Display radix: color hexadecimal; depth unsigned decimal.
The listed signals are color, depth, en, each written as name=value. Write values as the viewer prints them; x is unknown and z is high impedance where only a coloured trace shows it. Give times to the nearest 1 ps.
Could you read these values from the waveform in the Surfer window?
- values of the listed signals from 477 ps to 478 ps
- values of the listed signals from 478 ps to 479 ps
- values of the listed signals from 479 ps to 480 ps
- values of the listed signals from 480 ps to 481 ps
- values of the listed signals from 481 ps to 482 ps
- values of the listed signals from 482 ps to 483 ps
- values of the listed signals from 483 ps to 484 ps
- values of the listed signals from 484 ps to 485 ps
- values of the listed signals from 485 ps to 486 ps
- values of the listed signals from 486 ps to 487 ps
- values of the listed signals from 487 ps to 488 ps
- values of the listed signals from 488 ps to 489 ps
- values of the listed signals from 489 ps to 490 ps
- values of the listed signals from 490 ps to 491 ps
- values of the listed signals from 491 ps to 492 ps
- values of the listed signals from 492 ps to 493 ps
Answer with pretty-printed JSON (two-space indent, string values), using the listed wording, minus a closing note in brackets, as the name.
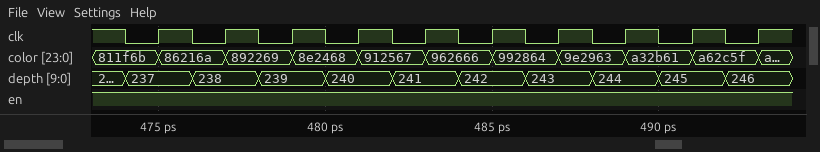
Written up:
{
  "values of the listed signals from 477 ps to 478 ps": "color=892269, depth=238, en=1",
  "values of the listed signals from 478 ps to 479 ps": "color=892269, depth=239, en=1",
  "values of the listed signals from 479 ps to 480 ps": "color=8e2468, depth=239, en=1",
  "values of the listed signals from 480 ps to 481 ps": "color=8e2468, depth=240, en=1",
  "values of the listed signals from 481 ps to 482 ps": "color=912567, depth=240, en=1",
  "values of the listed signals from 482 ps to 483 ps": "color=912567, depth=241, en=1",
  "values of the listed signals from 483 ps to 484 ps": "color=962666, depth=241, en=1",
  "values of the listed signals from 484 ps to 485 ps": "color=962666, depth=242, en=1",
  "values of the listed signals from 485 ps to 486 ps": "color=992864, depth=242, en=1",
  "values of the listed signals from 486 ps to 487 ps": "color=992864, depth=243, en=1",
  "values of the listed signals from 487 ps to 488 ps": "color=9e2963, depth=243, en=1",
  "values of the listed signals from 488 ps to 489 ps": "color=9e2963, depth=244, en=1",
  "values of the listed signals from 489 ps to 490 ps": "color=a32b61, depth=244, en=1",
  "values of the listed signals from 490 ps to 491 ps": "color=a32b61, depth=245, en=1",
  "values of the listed signals from 491 ps to 492 ps": "color=a62c5f, depth=245, en=1",
  "values of the listed signals from 492 ps to 493 ps": "color=a62c5f, depth=246, en=1"
}
